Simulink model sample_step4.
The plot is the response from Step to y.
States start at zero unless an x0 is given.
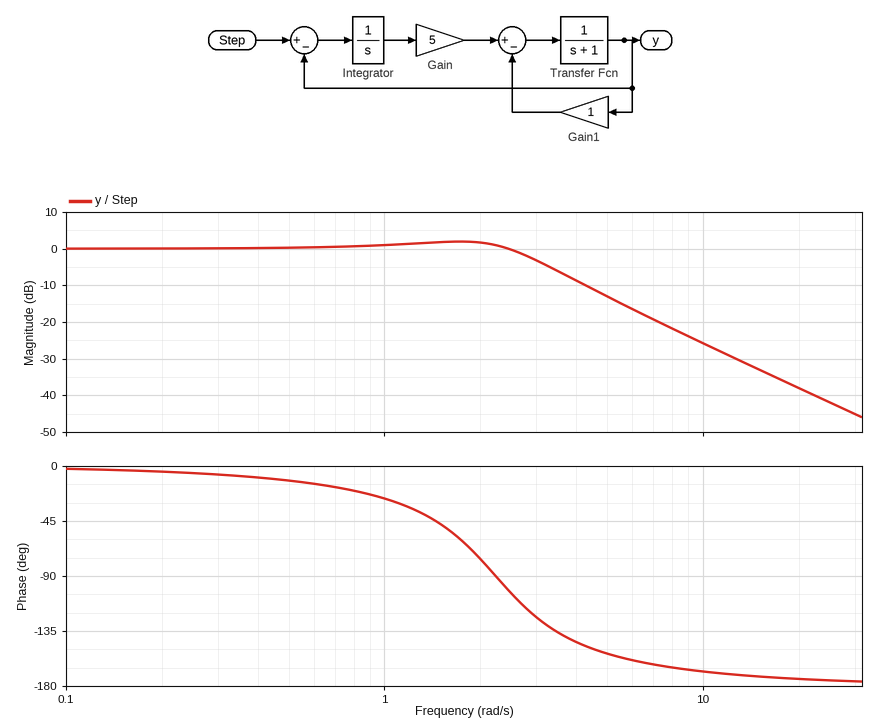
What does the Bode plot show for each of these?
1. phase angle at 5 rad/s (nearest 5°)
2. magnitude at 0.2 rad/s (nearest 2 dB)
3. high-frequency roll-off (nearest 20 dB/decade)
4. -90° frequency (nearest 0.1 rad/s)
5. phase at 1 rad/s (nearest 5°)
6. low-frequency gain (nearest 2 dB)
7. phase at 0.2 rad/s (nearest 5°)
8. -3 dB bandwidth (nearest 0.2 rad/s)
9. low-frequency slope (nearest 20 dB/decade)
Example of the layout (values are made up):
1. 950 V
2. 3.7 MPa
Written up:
1. -155°
2. 0 dB
3. -40 dB/decade
4. 2.2 rad/s
5. -25°
6. 0 dB
7. -5°
8. 3.0 rad/s
9. 0 dB/decade
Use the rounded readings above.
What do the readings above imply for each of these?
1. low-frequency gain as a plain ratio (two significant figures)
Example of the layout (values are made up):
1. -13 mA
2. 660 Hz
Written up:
1. 1.0
